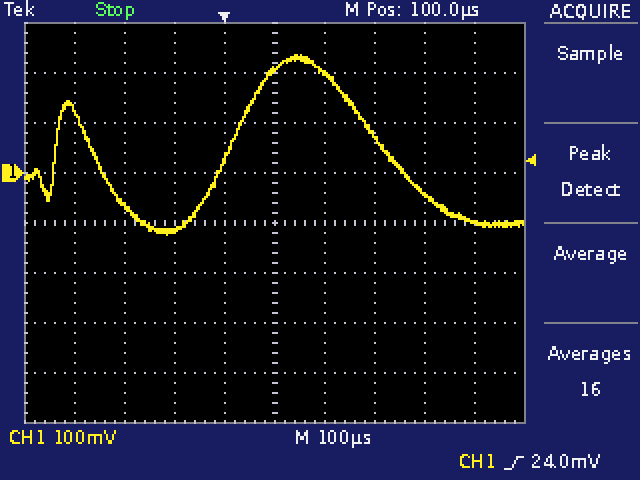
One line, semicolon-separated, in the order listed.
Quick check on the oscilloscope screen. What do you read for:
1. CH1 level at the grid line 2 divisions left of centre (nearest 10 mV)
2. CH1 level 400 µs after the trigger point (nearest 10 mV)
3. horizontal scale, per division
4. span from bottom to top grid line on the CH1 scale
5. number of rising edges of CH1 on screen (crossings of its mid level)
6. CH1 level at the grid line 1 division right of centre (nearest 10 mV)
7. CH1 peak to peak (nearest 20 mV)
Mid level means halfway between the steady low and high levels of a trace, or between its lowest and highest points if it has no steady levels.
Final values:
-110 mV; -40 mV; 100 µs; 800 mV; 2; 200 mV; 360 mV
